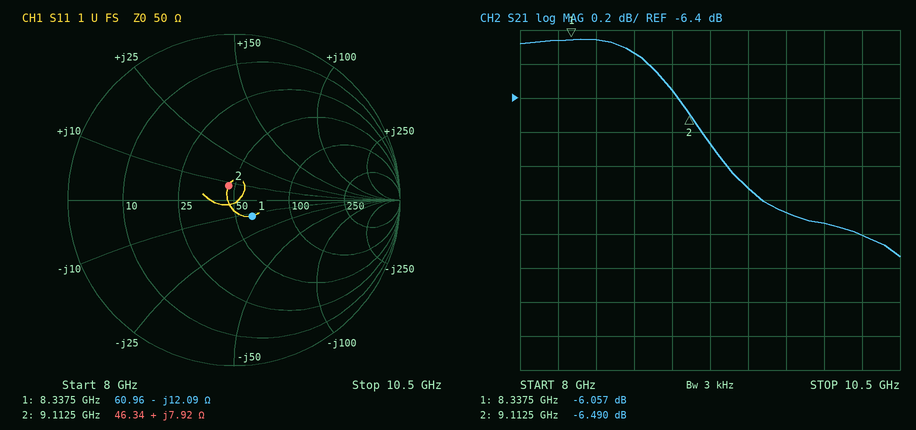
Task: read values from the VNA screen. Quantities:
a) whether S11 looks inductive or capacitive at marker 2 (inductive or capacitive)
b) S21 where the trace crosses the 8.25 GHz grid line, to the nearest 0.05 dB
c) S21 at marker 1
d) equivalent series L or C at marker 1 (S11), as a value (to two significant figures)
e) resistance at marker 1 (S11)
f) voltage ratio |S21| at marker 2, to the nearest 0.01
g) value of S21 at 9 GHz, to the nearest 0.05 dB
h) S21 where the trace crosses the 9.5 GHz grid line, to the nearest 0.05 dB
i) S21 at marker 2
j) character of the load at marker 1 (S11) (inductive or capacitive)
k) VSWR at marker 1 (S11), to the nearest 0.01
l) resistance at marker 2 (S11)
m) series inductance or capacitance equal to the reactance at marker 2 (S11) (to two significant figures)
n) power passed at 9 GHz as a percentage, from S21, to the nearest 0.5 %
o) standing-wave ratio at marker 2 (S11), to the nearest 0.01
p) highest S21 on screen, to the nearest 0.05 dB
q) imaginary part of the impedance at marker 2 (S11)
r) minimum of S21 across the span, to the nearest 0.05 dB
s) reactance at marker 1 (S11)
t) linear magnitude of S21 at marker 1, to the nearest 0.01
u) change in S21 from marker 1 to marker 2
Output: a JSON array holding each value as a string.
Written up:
["inductive", "-6.05 dB", "-6.057 dB", "1.6 pF", "60.96 Ω", "0.47", "-6.35 dB", "-6.95 dB", "-6.490 dB", "capacitive", "1.34", "46.34 Ω", "140 pH", "23.0 %", "1.20", "-6.05 dB", "+7.92 Ω", "-7.35 dB", "-12.09 Ω", "0.50", "-0.433 dB"]
